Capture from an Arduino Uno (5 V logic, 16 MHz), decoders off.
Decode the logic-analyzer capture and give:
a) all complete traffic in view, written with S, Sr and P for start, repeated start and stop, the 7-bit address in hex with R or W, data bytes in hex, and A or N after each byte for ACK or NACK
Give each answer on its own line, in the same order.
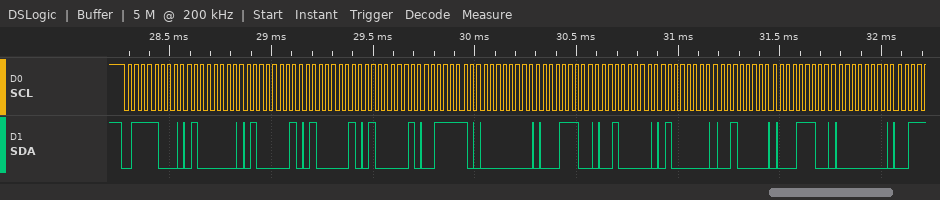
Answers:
S 3CW A 40 A 41 A 41 A 41 A 3E A 00 A 1C A 20 A 40 A 20 A 1C A 00 A
